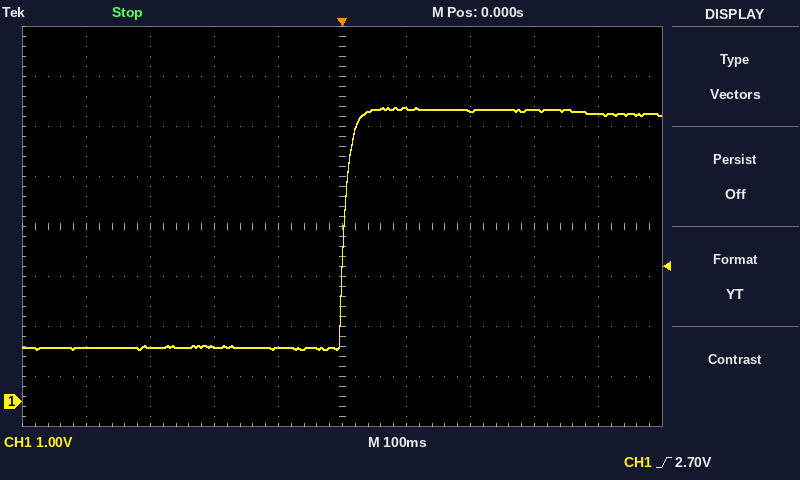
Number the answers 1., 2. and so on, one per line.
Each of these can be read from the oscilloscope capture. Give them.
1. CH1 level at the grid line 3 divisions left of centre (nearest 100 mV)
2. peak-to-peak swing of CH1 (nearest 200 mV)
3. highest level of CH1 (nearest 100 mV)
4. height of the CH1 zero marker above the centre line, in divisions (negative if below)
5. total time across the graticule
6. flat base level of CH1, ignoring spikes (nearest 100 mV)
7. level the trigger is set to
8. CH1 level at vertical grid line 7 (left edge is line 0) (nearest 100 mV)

1. 1.1 V
2. 4.8 V
3. 5.9 V
4. -3.5 div
5. 1 s
6. 1.1 V
7. 2.70 V
8. 5.8 V
